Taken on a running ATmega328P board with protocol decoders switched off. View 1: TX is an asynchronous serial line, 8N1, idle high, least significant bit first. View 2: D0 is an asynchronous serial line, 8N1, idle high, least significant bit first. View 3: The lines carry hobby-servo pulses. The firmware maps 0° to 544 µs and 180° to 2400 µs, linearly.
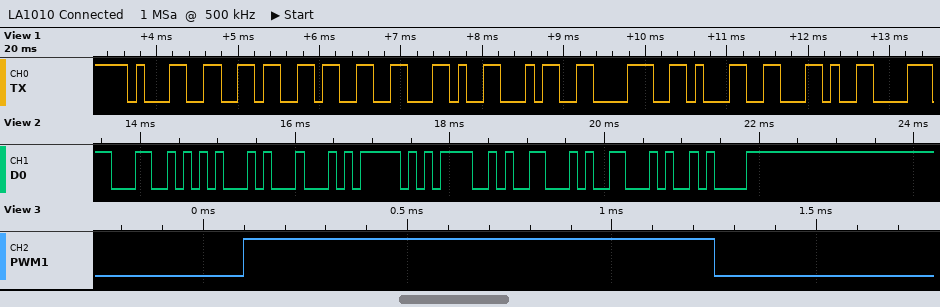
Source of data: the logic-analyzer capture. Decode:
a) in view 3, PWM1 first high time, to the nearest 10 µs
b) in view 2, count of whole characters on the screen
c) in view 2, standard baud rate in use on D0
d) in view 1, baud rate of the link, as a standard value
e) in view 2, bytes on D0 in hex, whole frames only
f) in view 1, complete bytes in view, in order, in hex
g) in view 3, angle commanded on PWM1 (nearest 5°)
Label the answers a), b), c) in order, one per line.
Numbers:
a) 1150 µs
b) 8
c) 9600 baud
d) 9600 baud
e) 4C 45 44 5F 4F 46 46 0A
f) 0x31 0x36 0x33 0x2C 0x34 0x38 0x31 0x2C
g) 60°
